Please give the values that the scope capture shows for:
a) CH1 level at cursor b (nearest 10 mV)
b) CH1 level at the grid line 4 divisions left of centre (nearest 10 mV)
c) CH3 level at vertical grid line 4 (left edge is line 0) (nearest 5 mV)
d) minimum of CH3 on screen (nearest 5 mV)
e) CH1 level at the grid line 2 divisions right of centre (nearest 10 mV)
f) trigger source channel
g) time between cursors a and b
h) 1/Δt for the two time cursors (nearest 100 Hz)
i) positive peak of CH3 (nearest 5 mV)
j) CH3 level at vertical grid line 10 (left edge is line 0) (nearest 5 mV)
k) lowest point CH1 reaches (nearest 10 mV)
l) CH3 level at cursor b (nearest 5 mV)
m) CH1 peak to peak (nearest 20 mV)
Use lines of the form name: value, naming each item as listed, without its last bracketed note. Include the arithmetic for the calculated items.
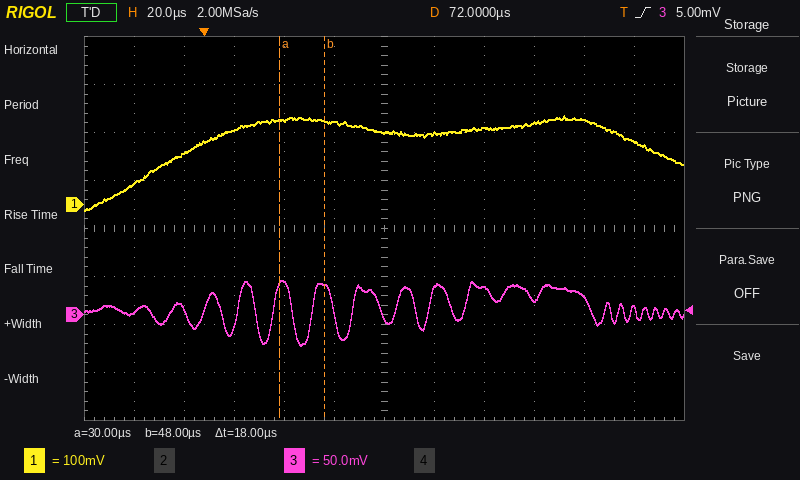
CH1 level at cursor b: 170 mV
CH1 level at the grid line 4 divisions left of centre: 110 mV
CH3 level at vertical grid line 4 (left edge is line 0): 35 mV
minimum of CH3 on screen: -30 mV
CH1 level at the grid line 2 divisions right of centre: 160 mV
trigger source channel: CH3
time between cursors a and b: 18 µs
1/Δt for the two time cursors: 1 / 18 µs ≈ 55.6 kHz
positive peak of CH3: 35 mV
CH3 level at vertical grid line 10 (left edge is line 0): 20 mV
lowest point CH1 reaches: -10 mV
CH3 level at cursor b: 30 mV
CH1 peak to peak: 200 mV
